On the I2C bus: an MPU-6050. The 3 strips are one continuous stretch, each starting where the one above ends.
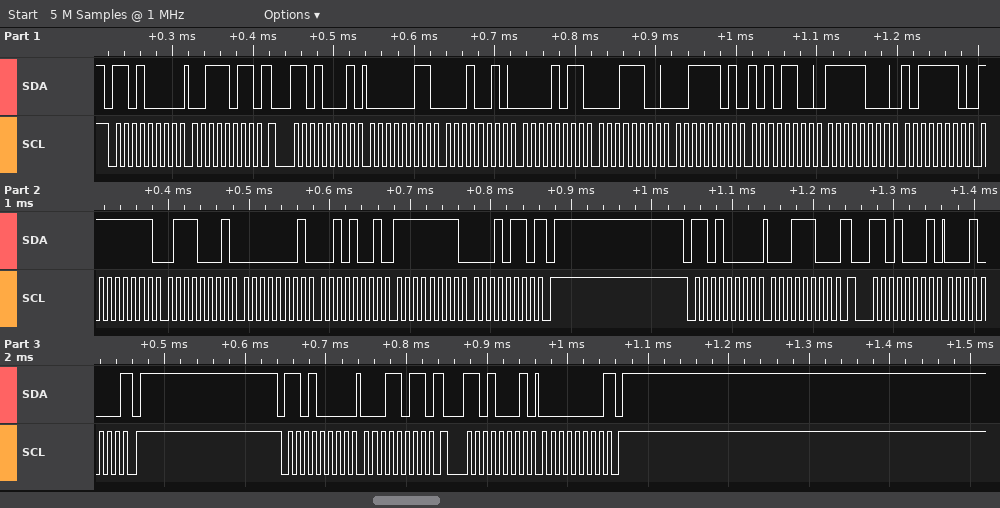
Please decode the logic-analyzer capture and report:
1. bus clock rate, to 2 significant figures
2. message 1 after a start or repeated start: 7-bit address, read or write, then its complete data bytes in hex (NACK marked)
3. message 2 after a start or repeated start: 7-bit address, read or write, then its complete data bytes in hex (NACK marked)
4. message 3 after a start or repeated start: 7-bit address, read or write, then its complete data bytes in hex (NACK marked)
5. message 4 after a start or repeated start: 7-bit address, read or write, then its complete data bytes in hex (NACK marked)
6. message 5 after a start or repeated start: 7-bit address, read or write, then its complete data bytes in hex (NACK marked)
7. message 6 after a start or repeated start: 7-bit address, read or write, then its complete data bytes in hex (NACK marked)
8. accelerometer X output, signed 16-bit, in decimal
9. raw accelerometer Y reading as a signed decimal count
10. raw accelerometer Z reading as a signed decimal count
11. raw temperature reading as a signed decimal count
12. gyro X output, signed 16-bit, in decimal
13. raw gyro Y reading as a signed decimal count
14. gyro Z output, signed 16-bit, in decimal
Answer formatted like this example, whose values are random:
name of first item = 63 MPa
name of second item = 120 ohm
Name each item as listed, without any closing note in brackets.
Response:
bus clock rate, to 2 significant figures = 100 kHz
message 1 after a start or repeated start: 7-bit address, read or write, then its complete data bytes in hex = 0x68 write: 3B
message 2 after a start or repeated start: 7-bit address, read or write, then its complete data bytes in hex = 0x68 read: 03 12 0B 1C 3D AC F8 BE FF 71 01 29 FF 16 NACK
message 3 after a start or repeated start: 7-bit address, read or write, then its complete data bytes in hex = 0x68 write: 1C
message 4 after a start or repeated start: 7-bit address, read or write, then its complete data bytes in hex = 0x68 read: 10 NACK
message 5 after a start or repeated start: 7-bit address, read or write, then its complete data bytes in hex = 0x68 write: 1B
message 6 after a start or repeated start: 7-bit address, read or write, then its complete data bytes in hex = 0x68 read: 00 NACK
accelerometer X output, signed 16-bit, in decimal = 786
raw accelerometer Y reading as a signed decimal count = 2844
raw accelerometer Z reading as a signed decimal count = 15788
raw temperature reading as a signed decimal count = -1858
gyro X output, signed 16-bit, in decimal = -143
raw gyro Y reading as a signed decimal count = 297
gyro Z output, signed 16-bit, in decimal = -234
